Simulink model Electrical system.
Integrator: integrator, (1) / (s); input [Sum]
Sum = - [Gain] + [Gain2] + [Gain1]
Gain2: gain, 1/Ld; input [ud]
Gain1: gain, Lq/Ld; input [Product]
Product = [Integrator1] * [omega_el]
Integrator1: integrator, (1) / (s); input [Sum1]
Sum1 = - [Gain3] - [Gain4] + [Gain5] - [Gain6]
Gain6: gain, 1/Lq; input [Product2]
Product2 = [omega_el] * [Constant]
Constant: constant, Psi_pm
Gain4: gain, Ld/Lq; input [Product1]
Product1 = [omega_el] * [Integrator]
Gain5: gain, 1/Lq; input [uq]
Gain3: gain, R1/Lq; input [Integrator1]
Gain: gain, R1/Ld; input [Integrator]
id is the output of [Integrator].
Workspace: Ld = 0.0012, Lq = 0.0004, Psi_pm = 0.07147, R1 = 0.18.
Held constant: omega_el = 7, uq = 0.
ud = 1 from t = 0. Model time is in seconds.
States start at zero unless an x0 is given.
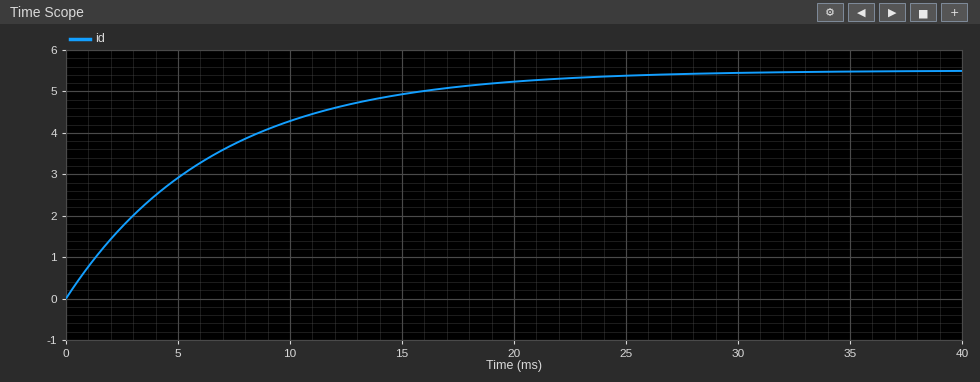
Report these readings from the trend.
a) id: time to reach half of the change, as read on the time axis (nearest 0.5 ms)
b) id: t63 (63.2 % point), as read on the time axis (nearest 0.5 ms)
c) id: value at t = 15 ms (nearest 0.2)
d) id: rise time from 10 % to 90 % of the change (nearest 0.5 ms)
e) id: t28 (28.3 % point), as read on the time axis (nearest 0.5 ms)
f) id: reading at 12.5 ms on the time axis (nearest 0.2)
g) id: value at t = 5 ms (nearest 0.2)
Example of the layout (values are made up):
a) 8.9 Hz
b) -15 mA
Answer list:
a) 4.5 ms
b) 6.5 ms
c) 5.0
d) 14.5 ms
e) 2.0 ms
f) 4.6
g) 3.0
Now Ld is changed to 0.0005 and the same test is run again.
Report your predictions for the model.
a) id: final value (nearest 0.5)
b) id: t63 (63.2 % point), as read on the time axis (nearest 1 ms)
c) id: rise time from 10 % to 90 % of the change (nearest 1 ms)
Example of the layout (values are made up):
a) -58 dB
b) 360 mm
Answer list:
a) 5.5
b) 3 ms
c) 6 ms
